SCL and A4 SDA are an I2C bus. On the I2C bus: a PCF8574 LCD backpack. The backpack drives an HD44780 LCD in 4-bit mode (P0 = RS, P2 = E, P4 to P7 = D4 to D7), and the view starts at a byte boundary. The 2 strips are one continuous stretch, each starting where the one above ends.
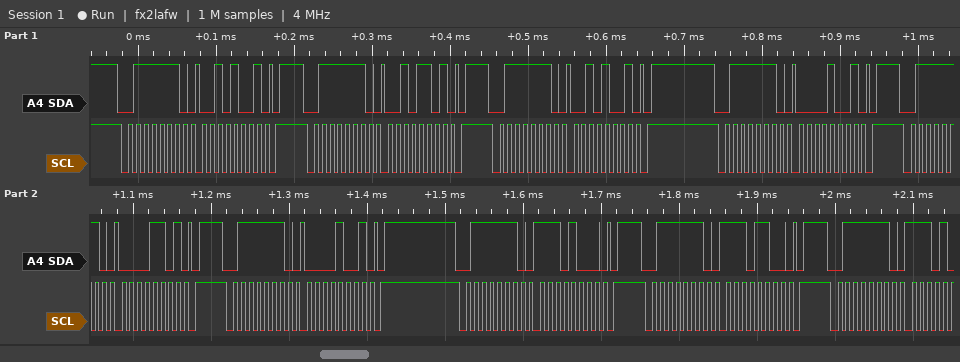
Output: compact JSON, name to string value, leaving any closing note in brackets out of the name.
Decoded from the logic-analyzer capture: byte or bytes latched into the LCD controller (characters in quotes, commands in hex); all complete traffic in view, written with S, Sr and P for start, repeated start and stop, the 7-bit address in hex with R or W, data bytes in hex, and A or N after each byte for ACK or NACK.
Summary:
{"byte or bytes latched into the LCD controller": "' '", "all complete traffic in view, written with S, Sr and P for start, repeated start and stop, the 7-bit address in hex with R or W, data bytes in hex, and A or N after each byte for ACK or NACK": "S 3FW A 29 A P S 3FW A 2D A P S 3FW A 29 A P S 3FW A 09 A P S 3FW A 0D A P S 3FW A 09 A P S 3FW A E8 A P S 3FW A EC A P S 3FW A"}
